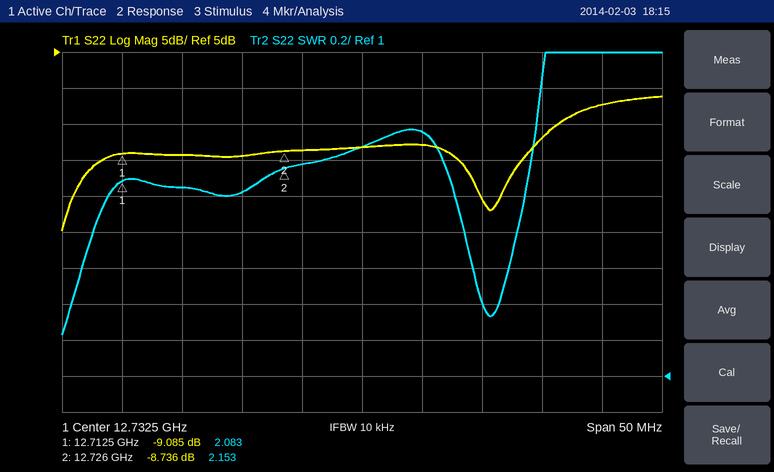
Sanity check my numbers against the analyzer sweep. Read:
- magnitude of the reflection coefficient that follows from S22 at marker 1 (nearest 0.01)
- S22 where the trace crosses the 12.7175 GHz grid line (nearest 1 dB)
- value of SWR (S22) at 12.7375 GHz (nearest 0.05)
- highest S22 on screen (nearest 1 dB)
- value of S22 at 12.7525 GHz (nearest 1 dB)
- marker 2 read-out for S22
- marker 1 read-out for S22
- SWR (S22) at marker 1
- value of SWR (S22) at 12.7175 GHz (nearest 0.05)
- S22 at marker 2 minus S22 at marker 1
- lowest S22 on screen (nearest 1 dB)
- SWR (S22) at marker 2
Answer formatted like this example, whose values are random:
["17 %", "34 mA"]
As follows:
["0.35", "-9 dB", "2.35", "-1 dB", "-2 dB", "-8.736 dB", "-9.085 dB", "2.083", "2.05", "0.349 dB", "-20 dB", "2.153"]
